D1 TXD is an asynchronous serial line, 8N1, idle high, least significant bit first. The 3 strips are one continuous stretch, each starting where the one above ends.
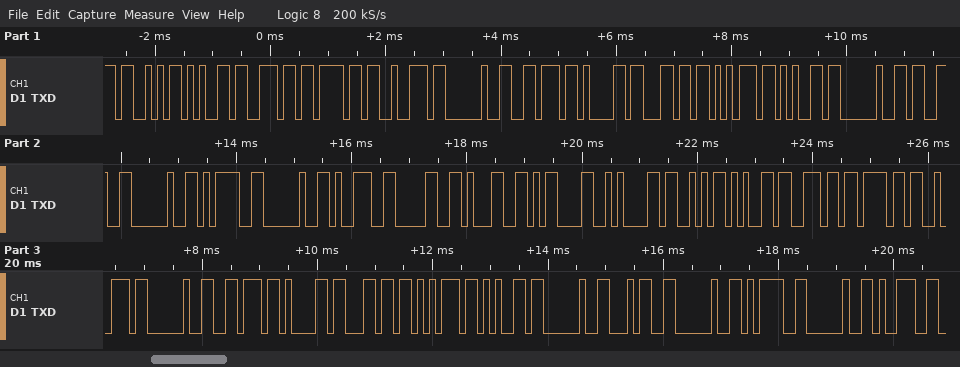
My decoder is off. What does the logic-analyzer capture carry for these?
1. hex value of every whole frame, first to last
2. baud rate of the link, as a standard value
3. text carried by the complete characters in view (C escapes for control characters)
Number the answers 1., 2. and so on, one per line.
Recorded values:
1. 53 65 6E 6F 72 20 76 61 6C 75 65 20 33 20 3D 20 39 30 31 0D 0A 53 65 6E 6F 72 20 76 61 6C 75 65 20 34 20 3D 20 39
2. 9600 baud
3. "Senor value 3 = 901\r\nSenor value 4 = 9"
